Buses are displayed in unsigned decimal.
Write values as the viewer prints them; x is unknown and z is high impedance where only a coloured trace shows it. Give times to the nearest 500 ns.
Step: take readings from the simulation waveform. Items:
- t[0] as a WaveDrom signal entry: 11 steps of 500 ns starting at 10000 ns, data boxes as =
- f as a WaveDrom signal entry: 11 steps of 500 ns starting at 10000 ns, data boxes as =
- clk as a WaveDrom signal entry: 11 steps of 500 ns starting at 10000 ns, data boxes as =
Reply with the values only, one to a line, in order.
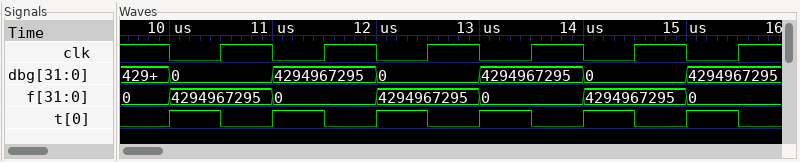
{name: 't[0]', wave: '10101010101'}
{name: 'f', wave: '=.=.=.=.=.=', data: '4294967295 0 4294967295 0 4294967295 0'}
{name: 'clk', wave: '01010101010'}
